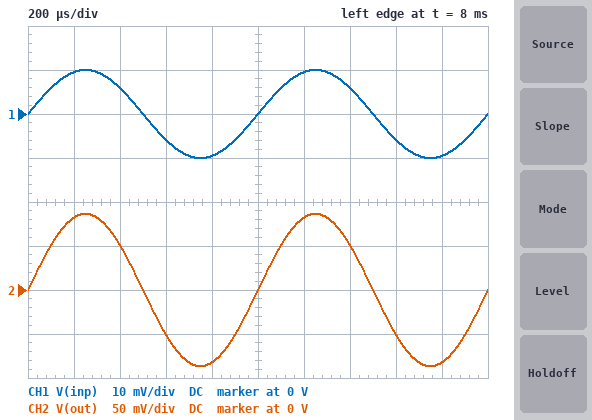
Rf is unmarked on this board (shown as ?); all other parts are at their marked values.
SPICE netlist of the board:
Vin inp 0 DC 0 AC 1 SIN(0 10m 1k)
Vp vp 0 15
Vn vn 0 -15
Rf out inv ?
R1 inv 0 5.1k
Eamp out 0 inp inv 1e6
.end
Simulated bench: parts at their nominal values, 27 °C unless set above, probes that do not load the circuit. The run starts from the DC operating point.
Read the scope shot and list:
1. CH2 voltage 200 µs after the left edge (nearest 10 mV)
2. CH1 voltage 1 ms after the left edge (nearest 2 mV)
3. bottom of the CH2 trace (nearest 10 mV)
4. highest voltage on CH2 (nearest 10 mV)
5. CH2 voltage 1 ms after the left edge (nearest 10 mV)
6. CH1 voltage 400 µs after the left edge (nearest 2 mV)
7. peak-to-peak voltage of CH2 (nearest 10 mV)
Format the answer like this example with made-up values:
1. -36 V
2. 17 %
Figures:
1. 80 mV
2. 0 V
3. -90 mV
4. 90 mV
5. 0 V
6. 6 mV
7. 170 mV
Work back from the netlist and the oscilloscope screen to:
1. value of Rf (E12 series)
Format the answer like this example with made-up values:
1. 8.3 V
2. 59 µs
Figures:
1. 39 kΩ
